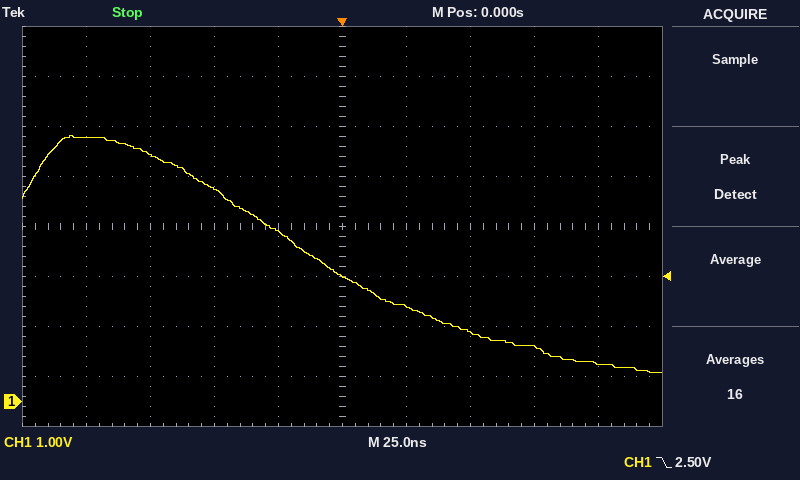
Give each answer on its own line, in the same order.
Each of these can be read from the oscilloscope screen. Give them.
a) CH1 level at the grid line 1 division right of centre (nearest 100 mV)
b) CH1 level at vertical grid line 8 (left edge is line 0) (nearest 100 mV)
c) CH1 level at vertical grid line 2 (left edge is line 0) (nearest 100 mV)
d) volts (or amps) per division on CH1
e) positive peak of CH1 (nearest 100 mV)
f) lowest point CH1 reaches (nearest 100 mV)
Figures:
1.9 V
1.1 V
4.9 V
1 V
5.3 V
600 mV
